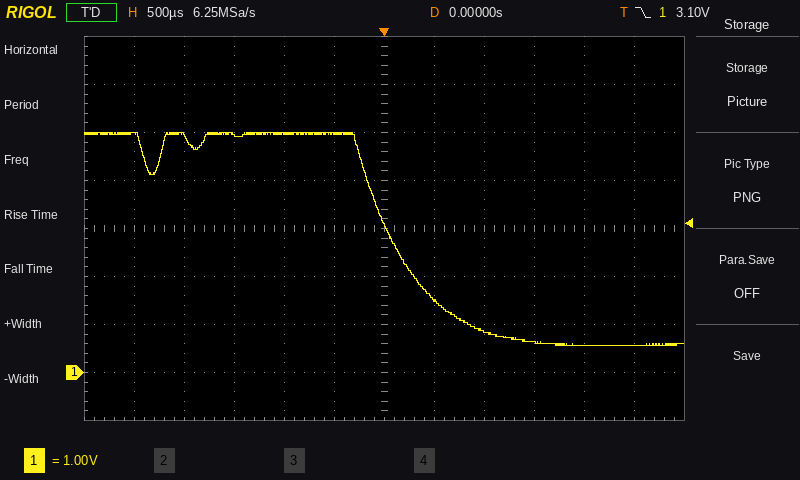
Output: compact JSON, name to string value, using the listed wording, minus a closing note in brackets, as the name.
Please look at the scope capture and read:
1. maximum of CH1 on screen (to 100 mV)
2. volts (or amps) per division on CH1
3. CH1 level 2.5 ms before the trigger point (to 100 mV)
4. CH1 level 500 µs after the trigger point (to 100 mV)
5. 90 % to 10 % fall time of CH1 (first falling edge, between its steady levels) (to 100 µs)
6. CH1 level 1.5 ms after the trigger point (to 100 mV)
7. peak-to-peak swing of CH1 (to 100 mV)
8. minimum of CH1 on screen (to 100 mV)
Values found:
{"maximum of CH1 on screen": "5.0 V", "volts (or amps) per division on CH1": "1 V", "CH1 level 2.5 ms before the trigger point": "5.0 V", "CH1 level 500 µs after the trigger point": "1.5 V", "90 % to 10 % fall time of CH1 (first falling edge, between its steady levels)": "1.1 ms", "CH1 level 1.5 ms after the trigger point": "600 mV", "peak-to-peak swing of CH1": "4.4 V", "minimum of CH1 on screen": "600 mV"}
